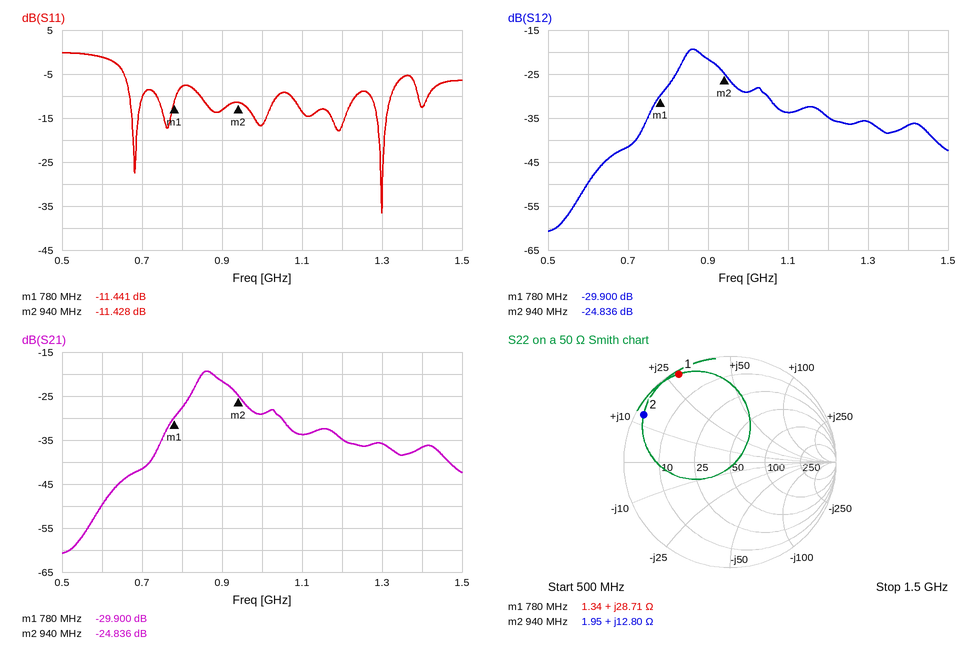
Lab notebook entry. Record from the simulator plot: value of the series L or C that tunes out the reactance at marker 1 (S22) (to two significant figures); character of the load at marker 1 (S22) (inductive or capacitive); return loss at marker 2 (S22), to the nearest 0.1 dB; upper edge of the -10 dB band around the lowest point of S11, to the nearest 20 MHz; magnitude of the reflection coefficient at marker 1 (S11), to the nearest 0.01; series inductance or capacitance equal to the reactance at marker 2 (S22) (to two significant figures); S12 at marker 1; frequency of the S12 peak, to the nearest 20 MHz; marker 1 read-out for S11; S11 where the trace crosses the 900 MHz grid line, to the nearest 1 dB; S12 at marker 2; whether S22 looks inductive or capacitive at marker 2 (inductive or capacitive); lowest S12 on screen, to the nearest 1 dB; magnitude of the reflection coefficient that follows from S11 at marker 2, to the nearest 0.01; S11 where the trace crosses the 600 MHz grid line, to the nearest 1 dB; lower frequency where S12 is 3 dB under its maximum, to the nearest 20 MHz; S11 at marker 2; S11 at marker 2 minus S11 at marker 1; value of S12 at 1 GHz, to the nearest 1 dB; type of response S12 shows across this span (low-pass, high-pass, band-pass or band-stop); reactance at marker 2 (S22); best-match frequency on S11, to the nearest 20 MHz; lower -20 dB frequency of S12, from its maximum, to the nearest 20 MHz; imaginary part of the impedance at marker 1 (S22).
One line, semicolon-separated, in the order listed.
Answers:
7.1 pF; inductive; 0.6 dB; 1.32 GHz; 0.27; 2.2 nH; -29.900 dB; 860 MHz; -11.441 dB; -13 dB; -24.836 dB; inductive; -61 dB; 0.27; -1 dB; 840 MHz; -11.428 dB; 0.013 dB; -29 dB; band-pass; +12.80 Ω; 1.30 GHz; 720 MHz; +28.71 Ω
